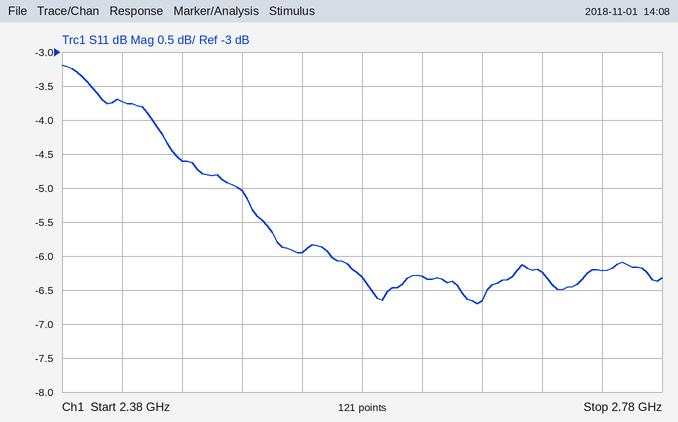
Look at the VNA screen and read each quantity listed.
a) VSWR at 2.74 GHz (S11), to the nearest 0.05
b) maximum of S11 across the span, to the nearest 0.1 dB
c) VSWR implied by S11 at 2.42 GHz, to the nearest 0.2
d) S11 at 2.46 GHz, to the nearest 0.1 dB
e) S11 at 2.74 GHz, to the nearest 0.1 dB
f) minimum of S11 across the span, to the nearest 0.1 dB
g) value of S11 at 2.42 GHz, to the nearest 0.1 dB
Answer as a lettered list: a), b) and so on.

a) 2.90
b) -3.2 dB
c) 4.8
d) -4.6 dB
e) -6.2 dB
f) -6.7 dB
g) -3.7 dB
